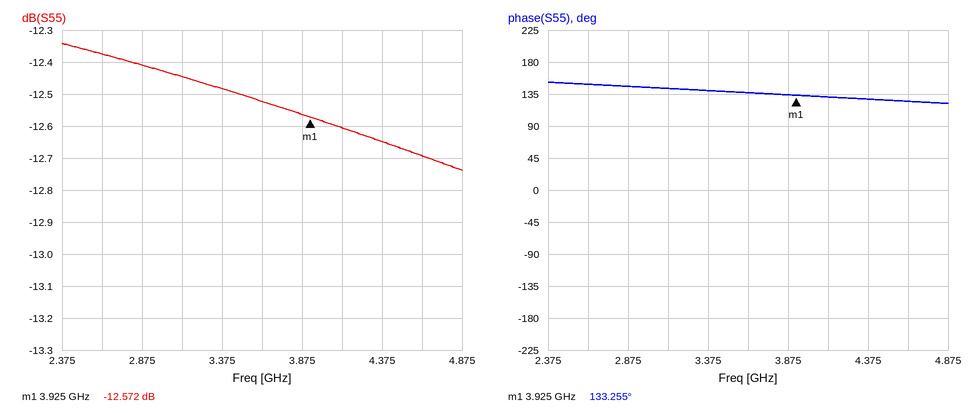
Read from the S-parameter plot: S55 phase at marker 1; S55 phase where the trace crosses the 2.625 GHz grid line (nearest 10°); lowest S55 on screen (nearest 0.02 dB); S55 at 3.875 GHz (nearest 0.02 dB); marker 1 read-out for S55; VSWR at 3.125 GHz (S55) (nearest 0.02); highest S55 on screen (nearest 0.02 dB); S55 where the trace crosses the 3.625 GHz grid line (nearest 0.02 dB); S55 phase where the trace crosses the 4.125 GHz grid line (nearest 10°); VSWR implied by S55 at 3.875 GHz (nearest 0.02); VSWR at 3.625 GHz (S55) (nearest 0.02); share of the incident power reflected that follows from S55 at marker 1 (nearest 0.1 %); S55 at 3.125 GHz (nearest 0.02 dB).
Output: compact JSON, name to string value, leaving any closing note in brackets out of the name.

{"S55 phase at marker 1": "133.255°", "S55 phase where the trace crosses the 2.625 GHz grid line": "150°", "lowest S55 on screen": "-12.74 dB", "S55 at 3.875 GHz": "-12.56 dB", "marker 1 read-out for S55": "-12.572 dB", "VSWR at 3.125 GHz (S55)": "1.62", "highest S55 on screen": "-12.34 dB", "S55 where the trace crosses the 3.625 GHz grid line": "-12.52 dB", "S55 phase where the trace crosses the 4.125 GHz grid line": "130°", "VSWR implied by S55 at 3.875 GHz": "1.62", "VSWR at 3.625 GHz (S55)": "1.62", "share of the incident power reflected that follows from S55 at marker 1": "5.5 %", "S55 at 3.125 GHz": "-12.44 dB"}
